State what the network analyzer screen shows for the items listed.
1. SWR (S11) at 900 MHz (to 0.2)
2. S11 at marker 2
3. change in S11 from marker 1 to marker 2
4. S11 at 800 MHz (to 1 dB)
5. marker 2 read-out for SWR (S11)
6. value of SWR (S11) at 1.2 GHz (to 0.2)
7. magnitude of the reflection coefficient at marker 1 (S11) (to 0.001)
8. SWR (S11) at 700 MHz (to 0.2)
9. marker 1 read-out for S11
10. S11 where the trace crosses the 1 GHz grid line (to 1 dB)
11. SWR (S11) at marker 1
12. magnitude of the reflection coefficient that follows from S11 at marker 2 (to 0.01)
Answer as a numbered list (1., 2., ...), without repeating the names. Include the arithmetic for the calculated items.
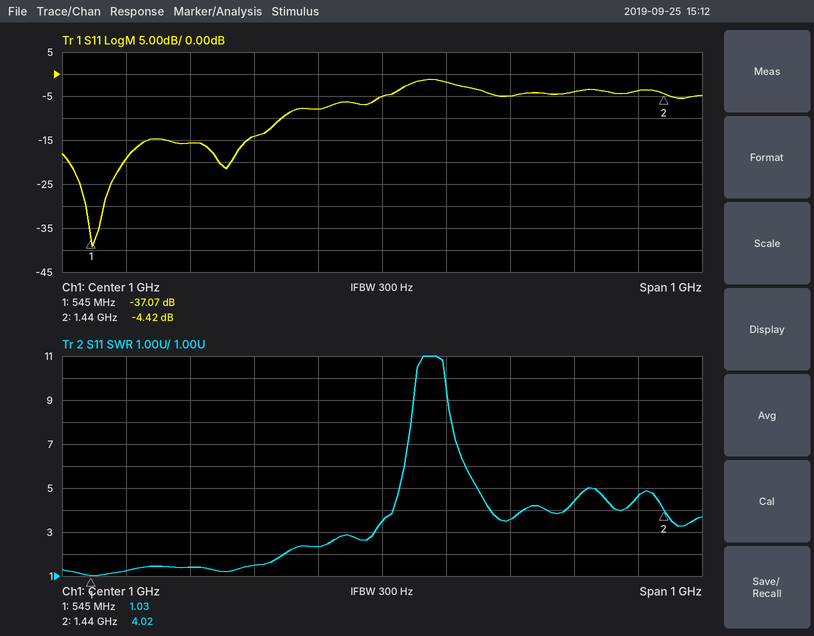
1. 2.4
2. -4.42 dB
3. -4.42 − (-37.07) = 32.65 dB
4. -14 dB
5. 4.02
6. 3.6
7. 10^(-37.07/20) ≈ 0.014
8. 1.4
9. -37.07 dB
10. -5 dB
11. 1.03
12. 10^(-4.42/20) ≈ 0.60
